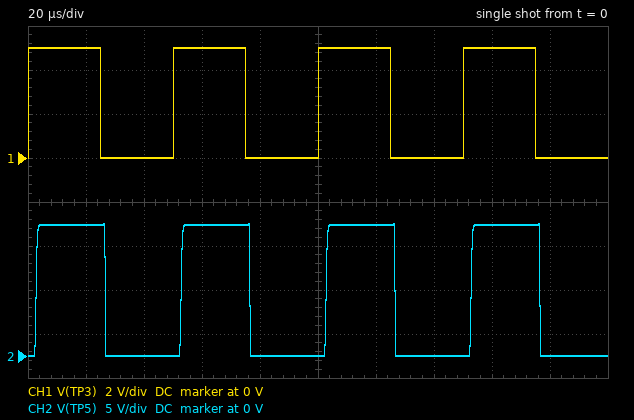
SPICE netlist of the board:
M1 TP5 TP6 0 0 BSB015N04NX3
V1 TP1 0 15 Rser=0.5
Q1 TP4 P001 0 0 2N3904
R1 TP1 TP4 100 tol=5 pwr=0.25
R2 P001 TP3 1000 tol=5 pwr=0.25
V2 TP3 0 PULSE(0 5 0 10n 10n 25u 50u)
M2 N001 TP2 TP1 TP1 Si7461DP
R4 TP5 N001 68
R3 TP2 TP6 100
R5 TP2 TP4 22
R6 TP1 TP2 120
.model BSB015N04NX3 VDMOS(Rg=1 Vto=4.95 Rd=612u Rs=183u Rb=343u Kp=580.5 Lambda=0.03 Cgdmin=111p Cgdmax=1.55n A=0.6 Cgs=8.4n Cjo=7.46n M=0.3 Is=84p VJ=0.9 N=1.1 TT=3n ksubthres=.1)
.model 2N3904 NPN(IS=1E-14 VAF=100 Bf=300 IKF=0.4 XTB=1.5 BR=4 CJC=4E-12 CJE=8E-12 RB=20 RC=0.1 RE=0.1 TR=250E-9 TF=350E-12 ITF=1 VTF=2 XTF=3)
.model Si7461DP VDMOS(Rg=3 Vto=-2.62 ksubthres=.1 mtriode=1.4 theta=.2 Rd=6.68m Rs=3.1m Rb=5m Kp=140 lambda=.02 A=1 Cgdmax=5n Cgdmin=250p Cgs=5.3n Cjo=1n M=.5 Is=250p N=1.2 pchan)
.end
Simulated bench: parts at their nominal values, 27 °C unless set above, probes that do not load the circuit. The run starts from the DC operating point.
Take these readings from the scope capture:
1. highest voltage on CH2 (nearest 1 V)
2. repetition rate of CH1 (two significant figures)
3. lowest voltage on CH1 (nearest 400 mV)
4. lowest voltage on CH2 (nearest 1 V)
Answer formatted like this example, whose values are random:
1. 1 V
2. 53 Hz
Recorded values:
1. 15 V
2. 20 kHz
3. 0 V
4. 0 V
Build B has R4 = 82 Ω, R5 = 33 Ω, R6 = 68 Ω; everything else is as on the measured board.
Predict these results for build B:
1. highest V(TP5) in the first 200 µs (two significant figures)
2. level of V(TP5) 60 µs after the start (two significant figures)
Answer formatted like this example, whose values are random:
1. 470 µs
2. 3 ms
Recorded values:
1. 5.4 mV
2. 5.2 mV
